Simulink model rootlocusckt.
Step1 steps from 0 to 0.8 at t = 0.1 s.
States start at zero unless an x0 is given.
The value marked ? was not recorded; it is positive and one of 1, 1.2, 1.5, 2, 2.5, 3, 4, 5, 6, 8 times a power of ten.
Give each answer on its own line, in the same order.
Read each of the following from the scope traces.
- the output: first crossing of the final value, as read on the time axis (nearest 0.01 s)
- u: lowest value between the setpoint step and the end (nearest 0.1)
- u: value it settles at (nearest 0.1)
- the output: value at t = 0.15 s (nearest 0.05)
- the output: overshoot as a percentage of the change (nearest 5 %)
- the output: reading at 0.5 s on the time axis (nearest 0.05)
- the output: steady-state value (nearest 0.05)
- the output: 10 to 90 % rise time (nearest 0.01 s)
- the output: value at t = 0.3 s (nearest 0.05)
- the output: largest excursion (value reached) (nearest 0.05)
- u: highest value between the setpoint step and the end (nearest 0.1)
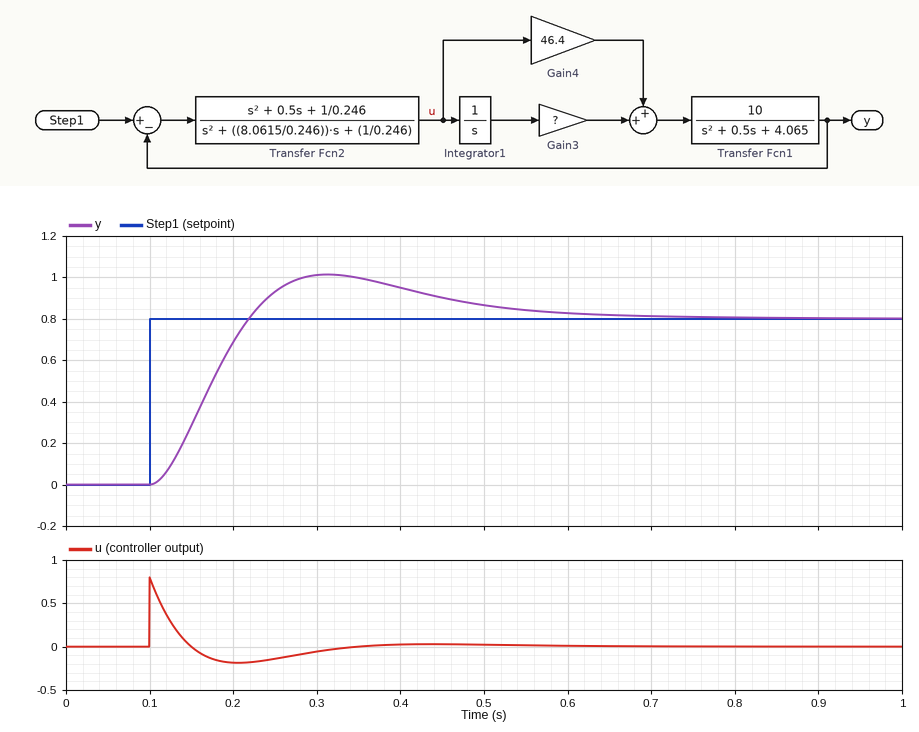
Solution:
0.22 s
-0.2
0.0
0.30
25 %
0.85
0.80
0.08 s
1.00
1.00
0.8
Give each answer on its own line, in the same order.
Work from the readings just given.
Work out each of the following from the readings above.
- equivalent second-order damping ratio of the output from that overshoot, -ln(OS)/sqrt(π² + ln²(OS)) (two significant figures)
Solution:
0.40
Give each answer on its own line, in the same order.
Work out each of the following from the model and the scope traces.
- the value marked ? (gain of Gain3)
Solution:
200
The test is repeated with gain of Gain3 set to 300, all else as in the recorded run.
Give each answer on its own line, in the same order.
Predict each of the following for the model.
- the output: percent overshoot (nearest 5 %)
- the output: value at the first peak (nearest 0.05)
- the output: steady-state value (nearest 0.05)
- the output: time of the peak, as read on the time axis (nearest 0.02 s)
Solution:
35 %
1.10
0.80
0.30 s
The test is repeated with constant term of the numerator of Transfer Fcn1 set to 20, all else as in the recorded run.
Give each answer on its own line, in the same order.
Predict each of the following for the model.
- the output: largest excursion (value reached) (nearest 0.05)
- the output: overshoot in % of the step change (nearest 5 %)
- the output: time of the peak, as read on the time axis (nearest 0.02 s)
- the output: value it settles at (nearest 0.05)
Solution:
1.05
30 %
0.22 s
0.80
